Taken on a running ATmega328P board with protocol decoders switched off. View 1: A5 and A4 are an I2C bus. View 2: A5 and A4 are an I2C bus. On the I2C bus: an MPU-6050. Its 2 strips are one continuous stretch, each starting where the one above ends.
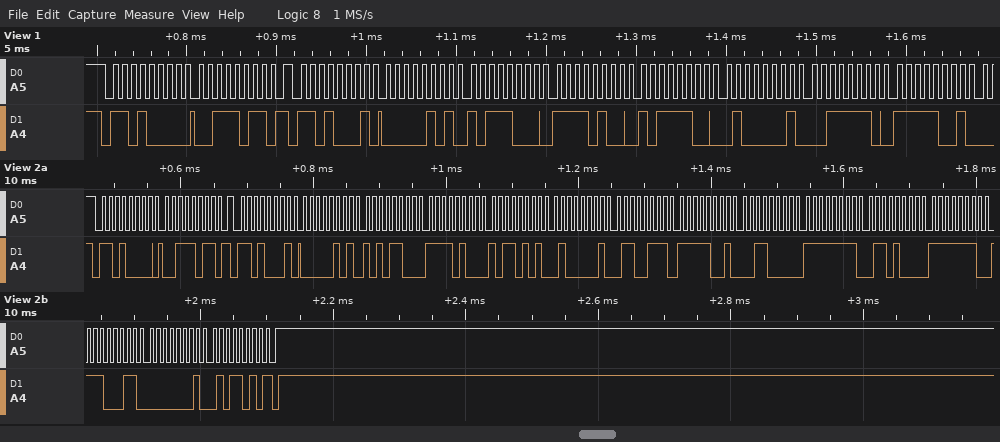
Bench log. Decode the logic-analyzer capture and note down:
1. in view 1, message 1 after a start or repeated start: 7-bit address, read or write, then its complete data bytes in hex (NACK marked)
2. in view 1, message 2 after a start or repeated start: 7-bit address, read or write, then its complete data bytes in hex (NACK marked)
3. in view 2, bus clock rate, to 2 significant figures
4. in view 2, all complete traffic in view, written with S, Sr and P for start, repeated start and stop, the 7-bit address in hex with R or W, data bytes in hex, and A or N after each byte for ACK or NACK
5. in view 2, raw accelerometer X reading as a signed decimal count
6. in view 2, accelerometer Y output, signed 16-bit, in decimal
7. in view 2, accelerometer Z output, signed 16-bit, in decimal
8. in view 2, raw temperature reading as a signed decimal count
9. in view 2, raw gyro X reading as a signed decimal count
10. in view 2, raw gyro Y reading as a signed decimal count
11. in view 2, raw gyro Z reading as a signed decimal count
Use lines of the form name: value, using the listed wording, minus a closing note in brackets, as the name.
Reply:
in view 1, message 1 after a start or repeated start: 7-bit address, read or write, then its complete data bytes in hex: 0x68 write: 3B
in view 1, message 2 after a start or repeated start: 7-bit address, read or write, then its complete data bytes in hex: 0x68 read: 05 B8 F4 BC 41 3E F9
in view 2, bus clock rate, to 2 significant figures: 100 kHz
in view 2, all complete traffic in view, written with S, Sr and P for start, repeated start and stop, the 7-bit address in hex with R or W, data bytes in hex, and A or N after each byte for ACK or NACK: S 68W A 3B A Sr 68R A 05 A AC A F4 A B5 A 41 A 67 A F9 A 30 A FF A 68 A FE A E3 A 01 A 5A N P
in view 2, raw accelerometer X reading as a signed decimal count: 1452
in view 2, accelerometer Y output, signed 16-bit, in decimal: -2891
in view 2, accelerometer Z output, signed 16-bit, in decimal: 16743
in view 2, raw temperature reading as a signed decimal count: -1744
in view 2, raw gyro X reading as a signed decimal count: -152
in view 2, raw gyro Y reading as a signed decimal count: -285
in view 2, raw gyro Z reading as a signed decimal count: 346
